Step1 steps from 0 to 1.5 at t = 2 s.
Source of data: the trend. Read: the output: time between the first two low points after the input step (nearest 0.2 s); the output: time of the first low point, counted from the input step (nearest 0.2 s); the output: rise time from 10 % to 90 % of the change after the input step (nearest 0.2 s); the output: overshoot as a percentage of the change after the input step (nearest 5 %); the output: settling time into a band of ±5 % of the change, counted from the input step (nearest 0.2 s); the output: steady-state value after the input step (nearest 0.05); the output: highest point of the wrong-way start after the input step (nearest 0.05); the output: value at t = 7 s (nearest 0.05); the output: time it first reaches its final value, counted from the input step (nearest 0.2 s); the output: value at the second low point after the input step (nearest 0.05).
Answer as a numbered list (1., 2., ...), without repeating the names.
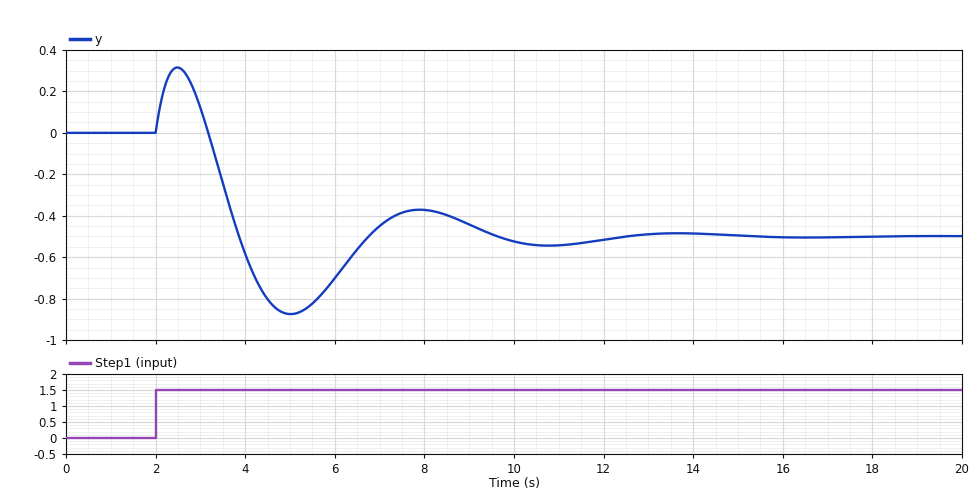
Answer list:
1. 5.8 s
2. 3.0 s
3. 0.6 s
4. 75 %
5. 9.8 s
6. -0.50
7. 0.30
8. -0.45
9. 1.8 s
10. -0.55
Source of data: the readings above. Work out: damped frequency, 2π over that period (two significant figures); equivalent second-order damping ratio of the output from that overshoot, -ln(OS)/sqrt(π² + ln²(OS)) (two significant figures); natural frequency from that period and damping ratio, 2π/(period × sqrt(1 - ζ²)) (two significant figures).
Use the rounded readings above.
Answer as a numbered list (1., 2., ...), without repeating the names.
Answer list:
1. 1.1 rad/s
2. 0.091
3. 1.1 rad/s
